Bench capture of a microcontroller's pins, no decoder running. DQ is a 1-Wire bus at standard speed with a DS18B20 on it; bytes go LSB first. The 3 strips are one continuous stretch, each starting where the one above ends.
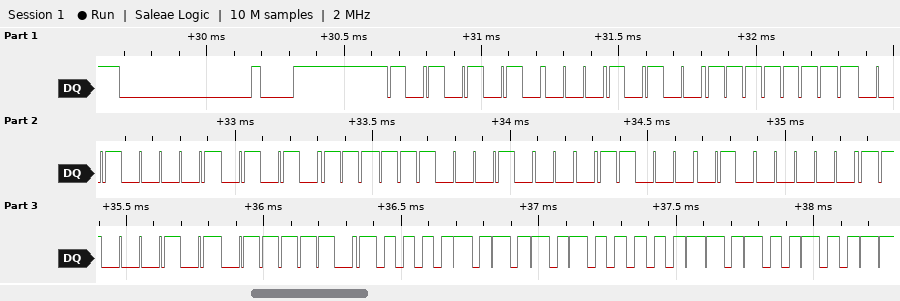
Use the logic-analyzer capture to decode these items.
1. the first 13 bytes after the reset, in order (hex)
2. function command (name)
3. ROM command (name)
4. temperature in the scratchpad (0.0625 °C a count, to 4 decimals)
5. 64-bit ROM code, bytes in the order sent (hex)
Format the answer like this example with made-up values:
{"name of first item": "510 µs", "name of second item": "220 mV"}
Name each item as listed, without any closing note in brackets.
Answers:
{"the first 13 bytes after the reset, in order": "55 28 FF 84 EA 47 18 02 A3 BE 50 05 4B", "function command": "Read Scratchpad", "ROM command": "Match ROM", "temperature in the scratchpad": "85.0000 °C", "64-bit ROM code, bytes in the order sent": "28 FF 84 EA 47 18 02 A3"}
